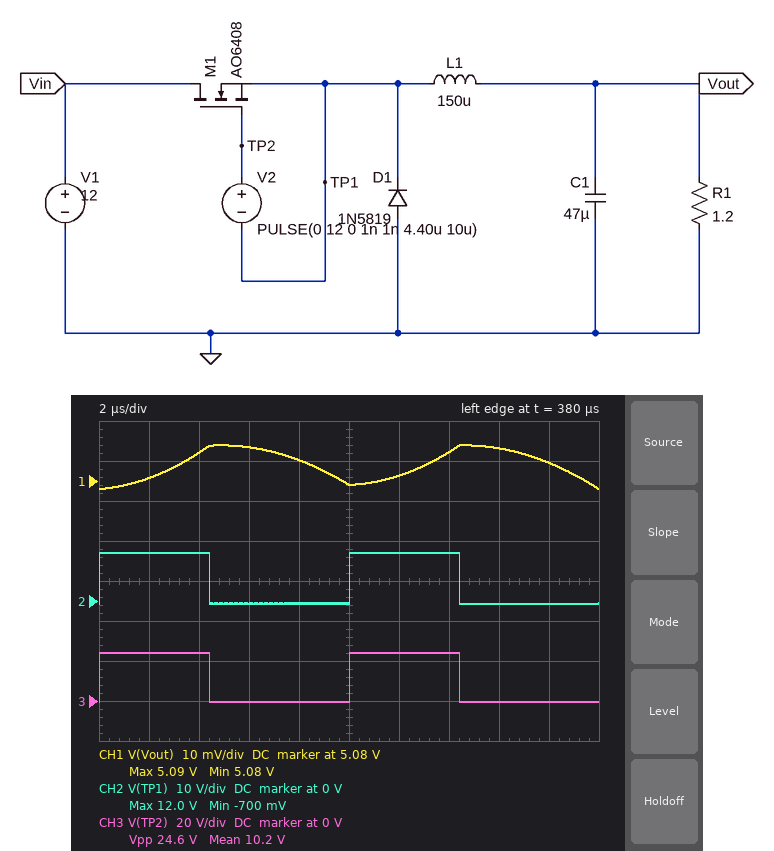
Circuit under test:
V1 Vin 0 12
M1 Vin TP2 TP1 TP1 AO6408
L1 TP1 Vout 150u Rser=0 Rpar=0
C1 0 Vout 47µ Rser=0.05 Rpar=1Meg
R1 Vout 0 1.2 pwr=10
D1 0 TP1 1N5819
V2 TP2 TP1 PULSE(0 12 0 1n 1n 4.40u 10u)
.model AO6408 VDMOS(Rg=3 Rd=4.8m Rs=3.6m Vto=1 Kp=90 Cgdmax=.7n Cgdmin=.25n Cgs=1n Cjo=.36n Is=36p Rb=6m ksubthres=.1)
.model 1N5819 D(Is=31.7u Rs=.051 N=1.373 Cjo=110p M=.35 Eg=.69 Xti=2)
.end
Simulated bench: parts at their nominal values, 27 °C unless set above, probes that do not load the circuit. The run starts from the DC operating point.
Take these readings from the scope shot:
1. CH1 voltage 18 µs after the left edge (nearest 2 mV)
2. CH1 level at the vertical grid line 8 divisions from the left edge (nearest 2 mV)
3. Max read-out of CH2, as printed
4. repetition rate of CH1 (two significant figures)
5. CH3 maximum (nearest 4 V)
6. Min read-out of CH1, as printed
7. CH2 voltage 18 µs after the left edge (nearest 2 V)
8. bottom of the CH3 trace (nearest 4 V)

5.084 V
5.088 V
12.0 V
100 kHz
24 V
5.08 V
0 V
0 V
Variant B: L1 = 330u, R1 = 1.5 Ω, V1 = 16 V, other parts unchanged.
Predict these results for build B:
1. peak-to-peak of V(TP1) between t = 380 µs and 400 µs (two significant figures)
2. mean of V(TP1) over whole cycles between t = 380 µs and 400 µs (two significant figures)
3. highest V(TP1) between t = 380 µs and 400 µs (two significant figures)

17 V
6.7 V
16 V
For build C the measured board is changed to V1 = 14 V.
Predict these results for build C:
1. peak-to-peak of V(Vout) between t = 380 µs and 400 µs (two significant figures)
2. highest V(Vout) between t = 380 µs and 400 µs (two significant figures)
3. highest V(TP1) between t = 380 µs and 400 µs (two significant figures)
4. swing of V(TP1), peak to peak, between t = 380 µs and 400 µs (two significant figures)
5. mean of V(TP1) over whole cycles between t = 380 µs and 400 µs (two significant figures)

13 mV
6.0 V
14 V
15 V
5.8 V
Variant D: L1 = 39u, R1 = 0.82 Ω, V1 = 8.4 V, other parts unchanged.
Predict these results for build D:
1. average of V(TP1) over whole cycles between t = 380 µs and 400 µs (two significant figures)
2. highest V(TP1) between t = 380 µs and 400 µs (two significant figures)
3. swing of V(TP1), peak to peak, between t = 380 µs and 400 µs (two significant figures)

3.3 V
8.4 V
9.0 V
